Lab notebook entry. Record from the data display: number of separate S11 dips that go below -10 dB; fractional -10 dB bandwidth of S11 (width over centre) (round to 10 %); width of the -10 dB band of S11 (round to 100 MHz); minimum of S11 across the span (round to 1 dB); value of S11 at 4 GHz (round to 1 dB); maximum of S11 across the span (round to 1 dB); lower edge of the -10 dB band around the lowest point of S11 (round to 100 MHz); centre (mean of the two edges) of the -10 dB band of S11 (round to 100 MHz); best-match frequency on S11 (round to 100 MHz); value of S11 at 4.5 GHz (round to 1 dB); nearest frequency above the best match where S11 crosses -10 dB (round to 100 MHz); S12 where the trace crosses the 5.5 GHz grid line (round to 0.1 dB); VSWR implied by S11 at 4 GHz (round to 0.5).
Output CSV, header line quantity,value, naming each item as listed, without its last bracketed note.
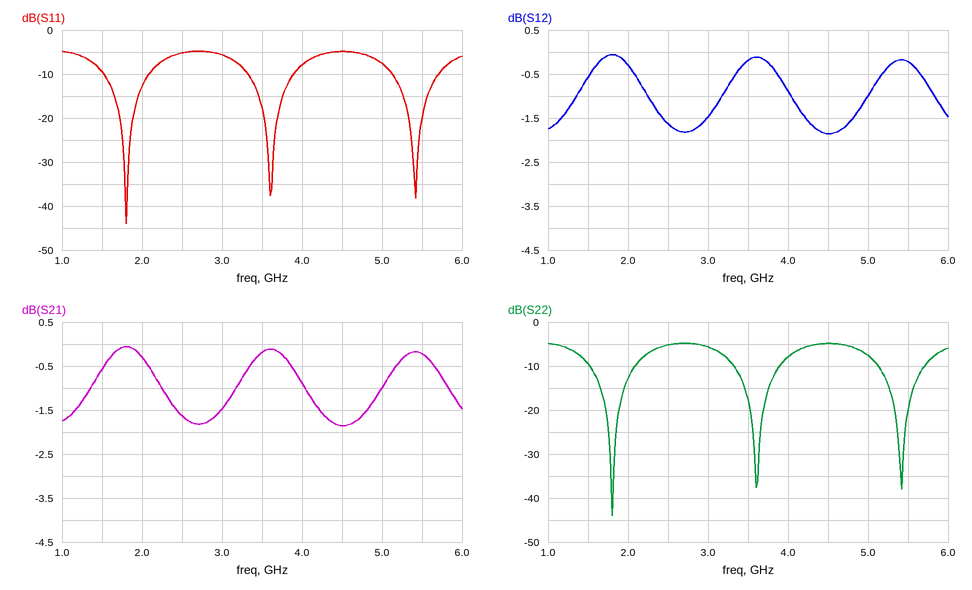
quantity,value
number of separate S11 dips that go below -10 dB,3
fractional -10 dB bandwidth of S11 (width over centre),30 %
width of the -10 dB band of S11,600 MHz
minimum of S11 across the span,-44 dB
value of S11 at 4 GHz,-8 dB
maximum of S11 across the span,-5 dB
lower edge of the -10 dB band around the lowest point of S11,1.5 GHz
centre (mean of the two edges) of the -10 dB band of S11,1.8 GHz
best-match frequency on S11,1.8 GHz
value of S11 at 4.5 GHz,-5 dB
nearest frequency above the best match where S11 crosses -10 dB,2.1 GHz
S12 where the trace crosses the 5.5 GHz grid line,-0.2 dB
VSWR implied by S11 at 4 GHz,2.5
